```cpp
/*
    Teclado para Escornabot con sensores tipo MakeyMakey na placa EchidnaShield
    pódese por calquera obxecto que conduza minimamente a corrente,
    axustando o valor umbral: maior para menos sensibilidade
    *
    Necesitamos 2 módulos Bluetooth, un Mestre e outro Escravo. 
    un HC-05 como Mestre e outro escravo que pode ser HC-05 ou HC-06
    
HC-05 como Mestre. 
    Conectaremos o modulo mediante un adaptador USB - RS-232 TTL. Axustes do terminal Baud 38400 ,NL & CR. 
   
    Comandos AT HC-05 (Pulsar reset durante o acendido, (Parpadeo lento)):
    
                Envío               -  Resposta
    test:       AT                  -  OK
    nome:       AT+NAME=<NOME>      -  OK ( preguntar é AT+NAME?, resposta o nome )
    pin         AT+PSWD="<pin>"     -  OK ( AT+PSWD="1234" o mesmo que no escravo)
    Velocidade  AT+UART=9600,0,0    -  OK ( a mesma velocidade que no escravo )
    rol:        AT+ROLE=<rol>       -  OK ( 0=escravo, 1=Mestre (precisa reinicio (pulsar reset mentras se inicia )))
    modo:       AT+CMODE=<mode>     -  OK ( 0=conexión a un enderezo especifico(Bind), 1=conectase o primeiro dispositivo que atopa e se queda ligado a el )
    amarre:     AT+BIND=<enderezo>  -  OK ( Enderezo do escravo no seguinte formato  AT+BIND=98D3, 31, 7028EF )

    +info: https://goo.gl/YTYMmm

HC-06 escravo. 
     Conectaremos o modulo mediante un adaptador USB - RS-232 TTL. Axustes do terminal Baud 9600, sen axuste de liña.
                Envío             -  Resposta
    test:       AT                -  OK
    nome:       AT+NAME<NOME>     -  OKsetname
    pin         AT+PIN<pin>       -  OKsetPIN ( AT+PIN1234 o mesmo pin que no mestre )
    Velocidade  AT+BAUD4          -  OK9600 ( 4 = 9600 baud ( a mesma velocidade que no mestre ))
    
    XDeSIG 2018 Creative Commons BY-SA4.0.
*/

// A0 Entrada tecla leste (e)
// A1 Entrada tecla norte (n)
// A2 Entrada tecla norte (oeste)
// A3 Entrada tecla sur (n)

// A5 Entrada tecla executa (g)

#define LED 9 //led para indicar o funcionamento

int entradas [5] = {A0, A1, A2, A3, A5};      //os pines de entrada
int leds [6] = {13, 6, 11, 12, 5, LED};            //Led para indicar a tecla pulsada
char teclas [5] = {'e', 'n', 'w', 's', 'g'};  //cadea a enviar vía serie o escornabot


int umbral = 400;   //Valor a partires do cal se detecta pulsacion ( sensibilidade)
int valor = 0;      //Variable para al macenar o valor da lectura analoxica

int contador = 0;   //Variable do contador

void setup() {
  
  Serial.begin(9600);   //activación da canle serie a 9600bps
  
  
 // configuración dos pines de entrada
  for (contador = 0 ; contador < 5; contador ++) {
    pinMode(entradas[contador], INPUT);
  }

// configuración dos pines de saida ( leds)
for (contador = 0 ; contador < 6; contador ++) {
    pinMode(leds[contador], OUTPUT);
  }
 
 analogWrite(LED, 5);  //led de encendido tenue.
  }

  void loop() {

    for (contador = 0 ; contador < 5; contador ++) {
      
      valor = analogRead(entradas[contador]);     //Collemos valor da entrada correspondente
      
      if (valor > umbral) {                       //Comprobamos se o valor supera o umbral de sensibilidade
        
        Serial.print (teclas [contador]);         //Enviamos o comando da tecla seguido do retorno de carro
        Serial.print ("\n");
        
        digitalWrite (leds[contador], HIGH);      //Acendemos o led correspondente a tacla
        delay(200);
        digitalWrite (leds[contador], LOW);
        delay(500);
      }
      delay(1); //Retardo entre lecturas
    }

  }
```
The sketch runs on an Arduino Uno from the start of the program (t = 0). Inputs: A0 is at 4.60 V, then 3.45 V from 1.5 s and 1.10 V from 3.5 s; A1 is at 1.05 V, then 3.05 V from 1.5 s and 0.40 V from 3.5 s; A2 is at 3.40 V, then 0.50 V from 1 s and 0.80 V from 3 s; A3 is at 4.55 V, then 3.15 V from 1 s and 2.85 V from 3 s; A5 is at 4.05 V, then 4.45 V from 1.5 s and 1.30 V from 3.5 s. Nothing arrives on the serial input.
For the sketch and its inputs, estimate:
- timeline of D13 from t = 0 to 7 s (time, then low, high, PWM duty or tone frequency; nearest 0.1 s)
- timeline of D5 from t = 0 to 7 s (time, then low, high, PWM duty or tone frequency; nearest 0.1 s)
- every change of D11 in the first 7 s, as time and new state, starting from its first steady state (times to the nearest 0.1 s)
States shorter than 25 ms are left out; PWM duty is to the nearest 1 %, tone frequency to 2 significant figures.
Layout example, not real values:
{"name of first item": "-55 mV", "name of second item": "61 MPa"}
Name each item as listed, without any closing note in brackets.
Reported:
{"timeline of D13 from t = 0 to 7 s": "0 s high; 0.2 s low; 2.8 s high; 3 s low", "timeline of D5 from t = 0 to 7 s": "0 s low; 2.1 s high; 2.3 s low", "every change of D11 in the first 7 s, as time and new state, starting from its first steady state": "0 s low; 0.7 s high; 0.9 s low"}
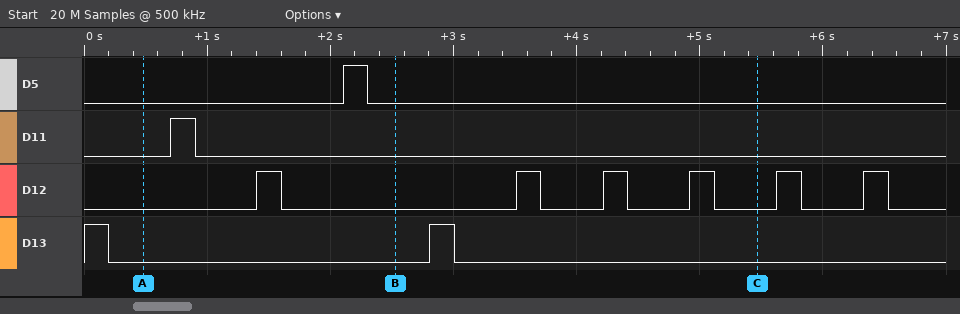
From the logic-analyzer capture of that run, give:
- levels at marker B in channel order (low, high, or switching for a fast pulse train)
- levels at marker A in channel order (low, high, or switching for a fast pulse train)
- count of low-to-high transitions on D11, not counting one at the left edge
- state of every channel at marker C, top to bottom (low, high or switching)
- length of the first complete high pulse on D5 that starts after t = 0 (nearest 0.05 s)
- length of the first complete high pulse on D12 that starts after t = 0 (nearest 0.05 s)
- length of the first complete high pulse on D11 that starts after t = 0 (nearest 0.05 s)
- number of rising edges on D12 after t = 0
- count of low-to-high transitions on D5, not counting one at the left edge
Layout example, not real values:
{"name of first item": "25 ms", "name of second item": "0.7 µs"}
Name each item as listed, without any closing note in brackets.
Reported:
{"levels at marker B in channel order": "D5 low, D11 low, D12 low, D13 low", "levels at marker A in channel order": "D5 low, D11 low, D12 low, D13 low", "count of low-to-high transitions on D11, not counting one at the left edge": "1", "state of every channel at marker C, top to bottom": "D5 low, D11 low, D12 low, D13 low", "length of the first complete high pulse on D5 that starts after t = 0": "0.20 s", "length of the first complete high pulse on D12 that starts after t = 0": "0.20 s", "length of the first complete high pulse on D11 that starts after t = 0": "0.20 s", "number of rising edges on D12 after t = 0": "6", "count of low-to-high transitions on D5, not counting one at the left edge": "1"}
